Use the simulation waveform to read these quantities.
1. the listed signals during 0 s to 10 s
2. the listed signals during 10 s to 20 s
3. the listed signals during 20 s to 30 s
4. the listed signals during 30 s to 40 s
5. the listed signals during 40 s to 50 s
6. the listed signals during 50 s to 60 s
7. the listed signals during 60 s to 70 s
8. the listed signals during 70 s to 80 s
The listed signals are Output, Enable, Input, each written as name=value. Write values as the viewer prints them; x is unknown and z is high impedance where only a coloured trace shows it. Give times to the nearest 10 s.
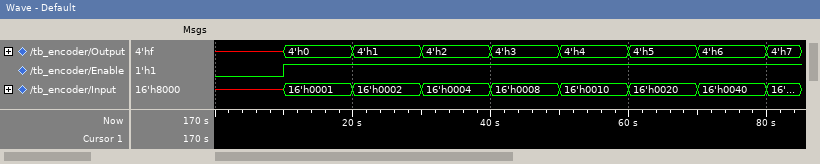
Output=x, Enable=0, Input=x
Output=4'h0, Enable=1, Input=16'h0001
Output=4'h1, Enable=1, Input=16'h0002
Output=4'h2, Enable=1, Input=16'h0004
Output=4'h3, Enable=1, Input=16'h0008
Output=4'h4, Enable=1, Input=16'h0010
Output=4'h5, Enable=1, Input=16'h0020
Output=4'h6, Enable=1, Input=16'h0040
